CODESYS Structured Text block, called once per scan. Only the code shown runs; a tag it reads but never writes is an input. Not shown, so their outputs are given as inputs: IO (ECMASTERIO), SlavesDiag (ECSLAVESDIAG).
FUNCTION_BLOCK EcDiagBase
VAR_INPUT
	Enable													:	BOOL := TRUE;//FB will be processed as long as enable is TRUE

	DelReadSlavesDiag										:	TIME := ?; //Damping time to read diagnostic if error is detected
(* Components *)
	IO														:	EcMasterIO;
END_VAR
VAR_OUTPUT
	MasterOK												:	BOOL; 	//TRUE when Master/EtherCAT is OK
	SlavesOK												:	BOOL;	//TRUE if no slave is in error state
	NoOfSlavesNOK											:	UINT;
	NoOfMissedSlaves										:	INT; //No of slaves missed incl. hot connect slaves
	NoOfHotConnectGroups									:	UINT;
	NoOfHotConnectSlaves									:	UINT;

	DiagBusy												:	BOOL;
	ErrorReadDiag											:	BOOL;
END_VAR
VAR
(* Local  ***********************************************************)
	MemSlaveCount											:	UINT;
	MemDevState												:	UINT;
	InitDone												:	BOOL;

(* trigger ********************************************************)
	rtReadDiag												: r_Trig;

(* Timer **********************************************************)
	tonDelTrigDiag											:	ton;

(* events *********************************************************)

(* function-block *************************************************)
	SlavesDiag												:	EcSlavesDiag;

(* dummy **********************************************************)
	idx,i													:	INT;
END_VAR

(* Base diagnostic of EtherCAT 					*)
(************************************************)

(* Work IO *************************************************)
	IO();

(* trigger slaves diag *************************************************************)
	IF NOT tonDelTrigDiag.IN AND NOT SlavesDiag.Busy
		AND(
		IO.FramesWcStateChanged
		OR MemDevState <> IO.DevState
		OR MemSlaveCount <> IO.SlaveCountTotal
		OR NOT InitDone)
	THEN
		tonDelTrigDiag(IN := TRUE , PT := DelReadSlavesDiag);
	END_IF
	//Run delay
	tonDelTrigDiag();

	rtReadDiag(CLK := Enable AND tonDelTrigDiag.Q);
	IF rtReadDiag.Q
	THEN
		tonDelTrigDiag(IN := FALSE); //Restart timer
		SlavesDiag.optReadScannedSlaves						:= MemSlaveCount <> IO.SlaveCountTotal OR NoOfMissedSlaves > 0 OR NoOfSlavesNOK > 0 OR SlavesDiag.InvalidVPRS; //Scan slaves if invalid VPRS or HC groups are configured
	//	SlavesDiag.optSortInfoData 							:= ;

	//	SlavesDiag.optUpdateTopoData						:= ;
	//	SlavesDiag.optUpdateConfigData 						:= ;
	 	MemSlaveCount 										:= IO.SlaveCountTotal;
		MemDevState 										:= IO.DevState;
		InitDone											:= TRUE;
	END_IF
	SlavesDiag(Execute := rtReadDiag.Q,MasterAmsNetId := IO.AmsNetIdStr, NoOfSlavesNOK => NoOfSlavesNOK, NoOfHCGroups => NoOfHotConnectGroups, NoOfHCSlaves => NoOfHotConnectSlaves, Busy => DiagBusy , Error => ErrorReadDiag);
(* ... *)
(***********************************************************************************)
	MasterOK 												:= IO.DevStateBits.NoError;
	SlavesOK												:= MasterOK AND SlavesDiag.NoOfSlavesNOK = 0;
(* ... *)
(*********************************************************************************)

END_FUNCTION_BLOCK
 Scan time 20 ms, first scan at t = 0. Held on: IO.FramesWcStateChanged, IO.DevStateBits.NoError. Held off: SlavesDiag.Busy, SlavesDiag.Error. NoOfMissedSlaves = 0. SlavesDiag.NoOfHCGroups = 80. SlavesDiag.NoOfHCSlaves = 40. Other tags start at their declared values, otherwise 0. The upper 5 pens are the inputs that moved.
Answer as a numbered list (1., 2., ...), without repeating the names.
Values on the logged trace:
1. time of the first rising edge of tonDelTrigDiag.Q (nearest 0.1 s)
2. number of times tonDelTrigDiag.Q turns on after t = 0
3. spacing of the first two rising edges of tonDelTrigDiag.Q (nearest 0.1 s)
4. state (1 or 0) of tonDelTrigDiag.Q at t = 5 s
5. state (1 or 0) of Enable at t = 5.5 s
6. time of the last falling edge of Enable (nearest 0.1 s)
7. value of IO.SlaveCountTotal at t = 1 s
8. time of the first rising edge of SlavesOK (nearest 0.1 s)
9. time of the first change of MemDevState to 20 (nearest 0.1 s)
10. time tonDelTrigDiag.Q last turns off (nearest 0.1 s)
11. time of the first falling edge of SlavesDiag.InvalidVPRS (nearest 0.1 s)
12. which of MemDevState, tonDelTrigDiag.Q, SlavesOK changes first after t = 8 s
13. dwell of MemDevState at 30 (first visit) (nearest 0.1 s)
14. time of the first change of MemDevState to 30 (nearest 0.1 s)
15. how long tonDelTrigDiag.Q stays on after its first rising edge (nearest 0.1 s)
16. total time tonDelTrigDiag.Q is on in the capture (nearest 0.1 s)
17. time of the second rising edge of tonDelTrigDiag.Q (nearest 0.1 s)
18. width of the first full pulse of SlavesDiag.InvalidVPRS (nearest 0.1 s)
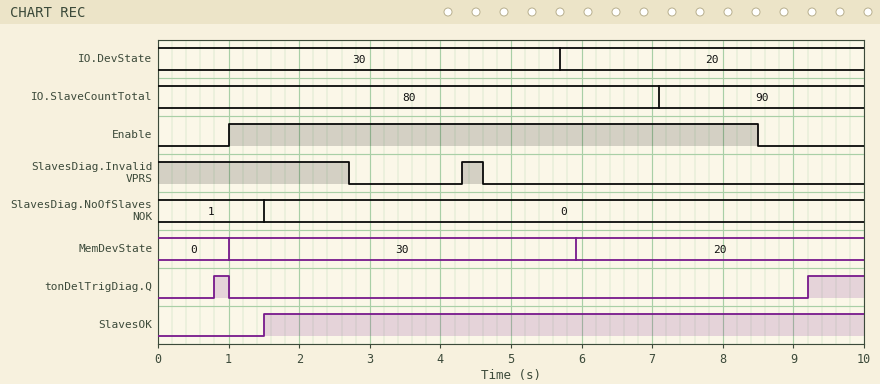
1. 0.8 s
2. 2
3. 8.4 s
4. 0
5. 1
6. 8.5 s
7. 80
8. 1.5 s
9. 5.9 s
10. 1.0 s
11. 2.7 s
12. tonDelTrigDiag.Q
13. 4.9 s
14. 1.0 s
15. 0.2 s
16. 1.0 s
17. 9.2 s
18. 0.3 s
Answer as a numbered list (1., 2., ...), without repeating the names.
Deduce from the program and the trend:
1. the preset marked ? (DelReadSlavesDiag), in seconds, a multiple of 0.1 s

1. 0.8 s
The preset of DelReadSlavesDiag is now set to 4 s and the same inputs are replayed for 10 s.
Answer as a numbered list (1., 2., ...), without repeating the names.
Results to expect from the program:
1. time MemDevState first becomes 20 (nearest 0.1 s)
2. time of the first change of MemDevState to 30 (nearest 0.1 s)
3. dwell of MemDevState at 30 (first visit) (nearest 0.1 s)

1. 8.0 s
2. 4.0 s
3. 4.0 s
